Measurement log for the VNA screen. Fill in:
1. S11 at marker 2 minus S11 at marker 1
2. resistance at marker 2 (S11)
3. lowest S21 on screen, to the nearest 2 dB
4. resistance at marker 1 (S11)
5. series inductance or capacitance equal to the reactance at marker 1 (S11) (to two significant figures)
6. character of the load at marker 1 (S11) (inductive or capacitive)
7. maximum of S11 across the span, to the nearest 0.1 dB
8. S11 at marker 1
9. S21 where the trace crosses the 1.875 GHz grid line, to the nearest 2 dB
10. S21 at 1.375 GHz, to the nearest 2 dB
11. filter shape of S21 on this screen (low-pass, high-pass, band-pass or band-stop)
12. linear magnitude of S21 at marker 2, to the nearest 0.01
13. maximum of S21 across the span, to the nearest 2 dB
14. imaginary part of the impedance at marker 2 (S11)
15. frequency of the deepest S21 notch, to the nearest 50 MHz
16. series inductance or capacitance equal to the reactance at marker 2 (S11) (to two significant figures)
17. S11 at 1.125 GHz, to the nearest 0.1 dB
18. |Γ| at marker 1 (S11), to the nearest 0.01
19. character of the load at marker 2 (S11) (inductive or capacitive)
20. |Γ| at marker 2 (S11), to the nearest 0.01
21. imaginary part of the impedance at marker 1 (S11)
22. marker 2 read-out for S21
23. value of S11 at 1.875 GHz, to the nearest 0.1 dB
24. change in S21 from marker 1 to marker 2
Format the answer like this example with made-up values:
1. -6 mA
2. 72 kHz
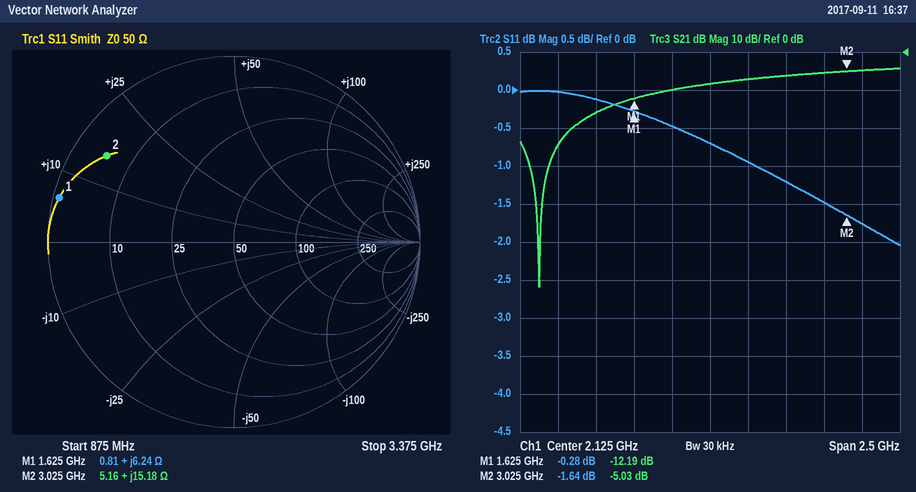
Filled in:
1. -1.36 dB
2. 5.16 Ω
3. -62 dB
4. 0.81 Ω
5. 610 pH
6. inductive
7. 0.0 dB
8. -0.28 dB
9. -10 dB
10. -16 dB
11. high-pass
12. 0.56
13. -4 dB
14. +15.18 Ω
15. 1.00 GHz
16. 800 pH
17. 0.0 dB
18. 0.97
19. inductive
20. 0.83
21. +6.24 Ω
22. -5.03 dB
23. -0.5 dB
24. 7.16 dB
